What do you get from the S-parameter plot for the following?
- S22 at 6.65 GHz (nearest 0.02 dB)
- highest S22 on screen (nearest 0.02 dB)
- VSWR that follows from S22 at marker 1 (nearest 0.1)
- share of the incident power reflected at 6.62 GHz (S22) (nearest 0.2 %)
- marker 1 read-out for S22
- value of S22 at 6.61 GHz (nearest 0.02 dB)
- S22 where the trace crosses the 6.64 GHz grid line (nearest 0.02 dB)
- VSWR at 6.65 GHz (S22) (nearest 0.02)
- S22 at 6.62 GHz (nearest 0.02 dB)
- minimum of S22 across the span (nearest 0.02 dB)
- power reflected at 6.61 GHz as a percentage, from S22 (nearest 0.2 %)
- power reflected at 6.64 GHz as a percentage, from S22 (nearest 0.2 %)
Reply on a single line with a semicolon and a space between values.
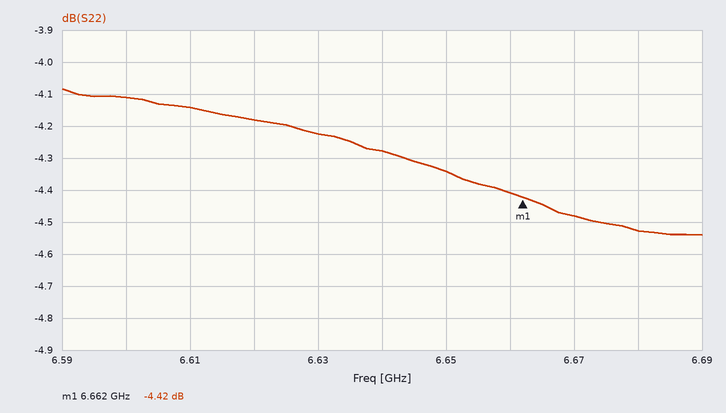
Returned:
-4.34 dB; -4.08 dB; 4.0; 38.2 %; -4.42 dB; -4.14 dB; -4.28 dB; 4.08; -4.18 dB; -4.54 dB; 38.6 %; 37.4 %
